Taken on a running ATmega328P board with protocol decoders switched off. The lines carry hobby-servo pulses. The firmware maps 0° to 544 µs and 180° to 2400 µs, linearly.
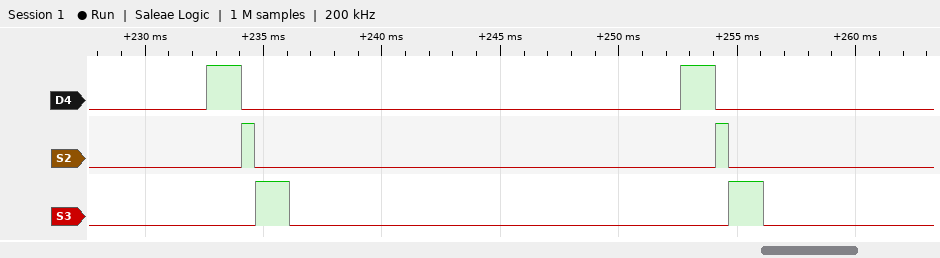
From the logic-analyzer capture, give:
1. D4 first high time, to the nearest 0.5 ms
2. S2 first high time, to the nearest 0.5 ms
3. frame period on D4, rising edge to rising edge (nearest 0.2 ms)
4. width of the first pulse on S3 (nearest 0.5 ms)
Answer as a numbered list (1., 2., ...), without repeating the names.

1. 1.5 ms
2. 0.5 ms
3. 20.0 ms
4. 1.5 ms
